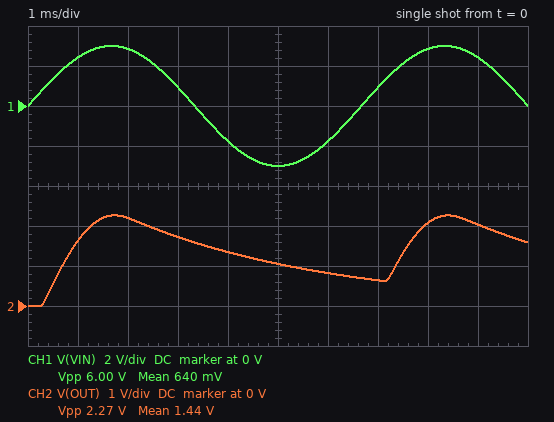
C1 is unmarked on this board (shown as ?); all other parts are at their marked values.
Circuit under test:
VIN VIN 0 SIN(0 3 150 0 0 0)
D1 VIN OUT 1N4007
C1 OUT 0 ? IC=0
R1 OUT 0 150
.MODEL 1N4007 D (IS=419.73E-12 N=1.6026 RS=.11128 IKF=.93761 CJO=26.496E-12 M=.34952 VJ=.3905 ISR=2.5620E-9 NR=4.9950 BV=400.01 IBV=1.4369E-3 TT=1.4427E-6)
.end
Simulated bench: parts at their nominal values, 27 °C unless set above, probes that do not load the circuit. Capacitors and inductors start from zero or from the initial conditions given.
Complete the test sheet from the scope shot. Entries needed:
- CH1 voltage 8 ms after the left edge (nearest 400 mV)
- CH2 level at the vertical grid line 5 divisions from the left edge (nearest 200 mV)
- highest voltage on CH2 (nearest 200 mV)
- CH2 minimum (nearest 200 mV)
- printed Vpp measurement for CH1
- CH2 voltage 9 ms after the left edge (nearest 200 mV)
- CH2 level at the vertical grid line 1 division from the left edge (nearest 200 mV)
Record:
2.8 V
1.0 V
2.2 V
0 V
6.00 V
2.0 V
1.6 V
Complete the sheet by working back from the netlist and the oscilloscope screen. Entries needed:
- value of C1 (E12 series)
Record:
27 µF
